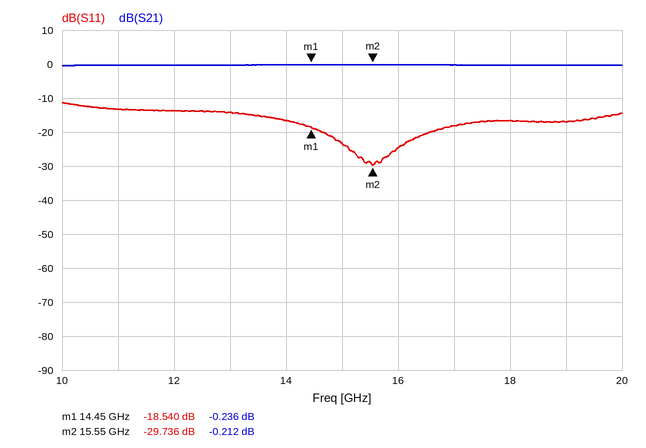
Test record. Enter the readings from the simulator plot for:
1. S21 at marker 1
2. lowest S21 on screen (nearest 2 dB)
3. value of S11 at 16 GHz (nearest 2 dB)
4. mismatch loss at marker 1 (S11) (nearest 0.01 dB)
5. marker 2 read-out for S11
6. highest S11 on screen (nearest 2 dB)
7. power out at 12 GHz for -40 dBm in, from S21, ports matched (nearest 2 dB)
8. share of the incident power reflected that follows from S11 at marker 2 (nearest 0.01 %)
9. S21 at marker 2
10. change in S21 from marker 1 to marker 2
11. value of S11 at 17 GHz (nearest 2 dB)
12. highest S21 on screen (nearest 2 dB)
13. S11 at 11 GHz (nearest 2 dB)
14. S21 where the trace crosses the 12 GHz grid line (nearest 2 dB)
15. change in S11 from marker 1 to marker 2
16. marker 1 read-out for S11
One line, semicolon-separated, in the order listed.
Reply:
-0.236 dB; 0 dB; -24 dB; 0.06 dB; -29.736 dB; -12 dB; -40 dBm; 0.11 %; -0.212 dB; 0.024 dB; -18 dB; 0 dB; -14 dB; 0 dB; -11.196 dB; -18.540 dB
